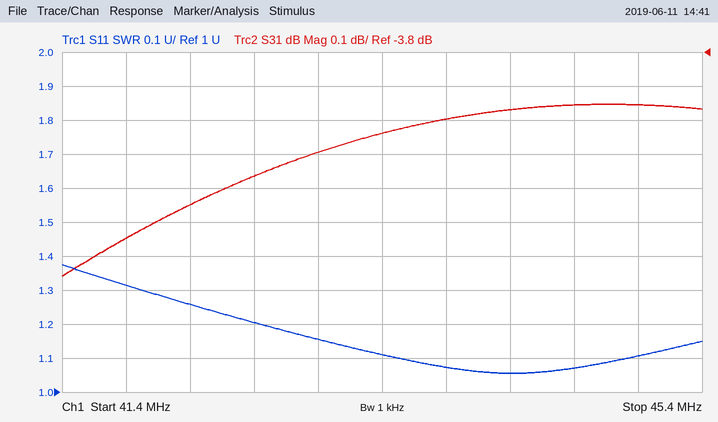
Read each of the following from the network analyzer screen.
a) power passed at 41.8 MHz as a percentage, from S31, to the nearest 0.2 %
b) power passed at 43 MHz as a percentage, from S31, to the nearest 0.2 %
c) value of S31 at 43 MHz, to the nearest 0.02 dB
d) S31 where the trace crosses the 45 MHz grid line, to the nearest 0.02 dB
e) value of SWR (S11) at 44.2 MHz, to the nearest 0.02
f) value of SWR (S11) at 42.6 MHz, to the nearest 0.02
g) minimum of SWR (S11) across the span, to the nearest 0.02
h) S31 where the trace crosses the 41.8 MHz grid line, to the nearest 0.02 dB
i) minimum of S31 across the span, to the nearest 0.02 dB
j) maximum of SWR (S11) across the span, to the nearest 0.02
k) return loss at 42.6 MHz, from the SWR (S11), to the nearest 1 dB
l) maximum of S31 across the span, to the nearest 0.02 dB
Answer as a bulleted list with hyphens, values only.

- 36.8 %
- 39.0 %
- -4.10 dB
- -3.96 dB
- 1.06
- 1.20
- 1.06
- -4.34 dB
- -4.46 dB
- 1.38
- 21 dB
- -3.96 dB
